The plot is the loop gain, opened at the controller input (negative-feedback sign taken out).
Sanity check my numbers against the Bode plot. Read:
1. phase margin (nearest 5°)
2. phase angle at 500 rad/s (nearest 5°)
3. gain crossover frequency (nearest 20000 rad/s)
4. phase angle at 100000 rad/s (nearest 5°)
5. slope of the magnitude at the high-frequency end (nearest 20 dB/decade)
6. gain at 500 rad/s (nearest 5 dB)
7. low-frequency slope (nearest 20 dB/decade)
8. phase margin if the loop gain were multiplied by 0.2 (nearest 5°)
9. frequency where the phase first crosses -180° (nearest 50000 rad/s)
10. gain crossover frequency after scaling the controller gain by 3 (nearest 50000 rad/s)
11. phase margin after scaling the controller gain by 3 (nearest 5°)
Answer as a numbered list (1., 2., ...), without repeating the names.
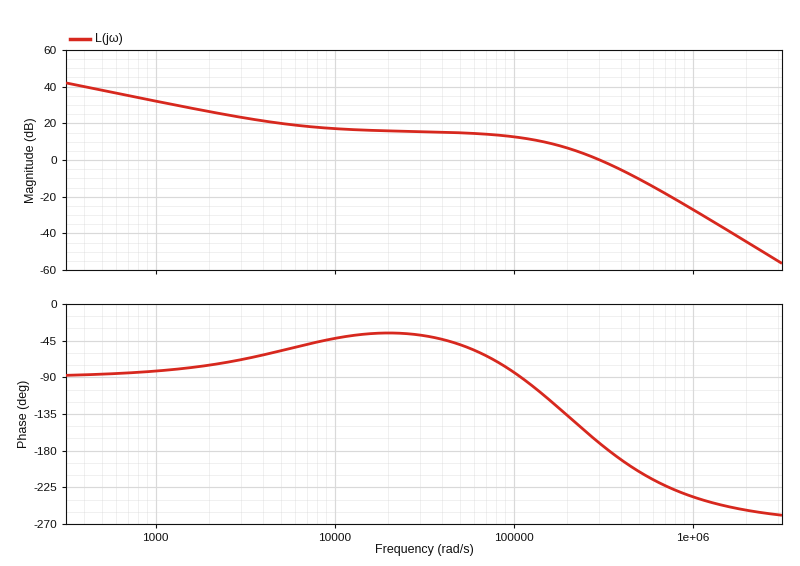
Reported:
1. 10°
2. -85°
3. 300000 rad/s
4. -85°
5. -60 dB/decade
6. 40 dB
7. -20 dB/decade
8. 115°
9. 350000 rad/s
10. 500000 rad/s
11. -25°
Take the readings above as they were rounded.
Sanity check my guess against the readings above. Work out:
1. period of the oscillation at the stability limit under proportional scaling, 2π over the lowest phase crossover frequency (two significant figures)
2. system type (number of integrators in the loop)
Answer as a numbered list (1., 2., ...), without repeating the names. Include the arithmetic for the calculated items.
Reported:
1. 2π / 350000 = 0.000018 s
2. 1
